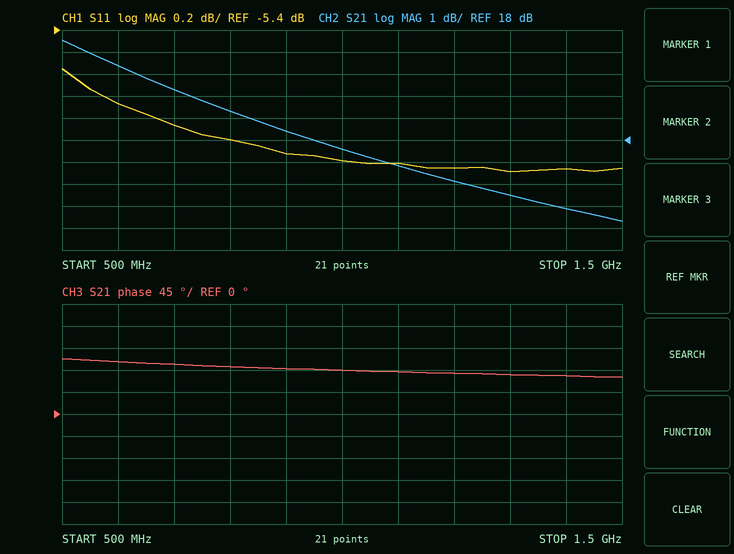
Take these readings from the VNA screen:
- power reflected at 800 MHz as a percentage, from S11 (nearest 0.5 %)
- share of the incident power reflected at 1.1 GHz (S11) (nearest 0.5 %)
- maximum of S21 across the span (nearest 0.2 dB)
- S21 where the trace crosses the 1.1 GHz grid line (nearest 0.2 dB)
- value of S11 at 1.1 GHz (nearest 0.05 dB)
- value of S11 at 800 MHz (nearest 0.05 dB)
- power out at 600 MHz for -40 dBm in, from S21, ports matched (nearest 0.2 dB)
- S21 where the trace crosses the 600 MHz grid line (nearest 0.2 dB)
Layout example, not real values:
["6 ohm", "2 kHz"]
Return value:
["23.0 %", "22.0 %", "22.6 dB", "16.8 dB", "-6.60 dB", "-6.40 dB", "-18.6 dBm", "21.4 dB"]
